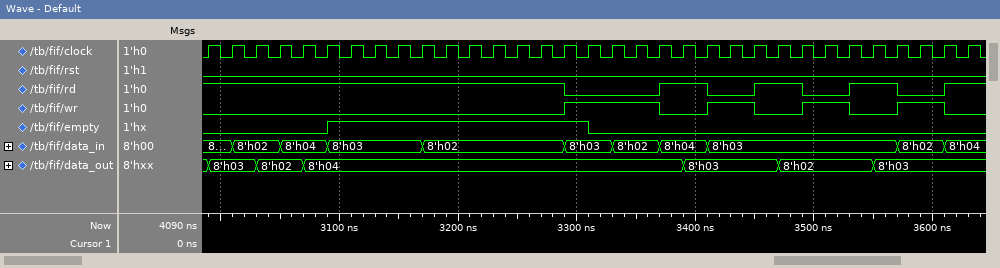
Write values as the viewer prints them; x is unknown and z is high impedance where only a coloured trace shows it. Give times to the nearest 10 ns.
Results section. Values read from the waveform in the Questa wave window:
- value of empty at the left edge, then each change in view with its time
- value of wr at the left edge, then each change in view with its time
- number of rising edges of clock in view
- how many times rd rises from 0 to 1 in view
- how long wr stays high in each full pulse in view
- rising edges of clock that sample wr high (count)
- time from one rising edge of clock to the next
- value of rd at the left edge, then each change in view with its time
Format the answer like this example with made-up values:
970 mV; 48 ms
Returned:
0, 1 at 3090 ns, 0 at 3310 ns; 0, 1 at 3290 ns, 0 at 3370 ns, 1 at 3410 ns, 0 at 3450 ns, 1 at 3490 ns, 0 at 3530 ns, 1 at 3570 ns, 0 at 3610 ns; 33; 4; 80 ns, 40 ns, 40 ns, 40 ns; 10; 20 ns; 1, 0 at 3290 ns, 1 at 3370 ns, 0 at 3410 ns, 1 at 3450 ns, 0 at 3490 ns, 1 at 3530 ns, 0 at 3570 ns, 1 at 3610 ns
